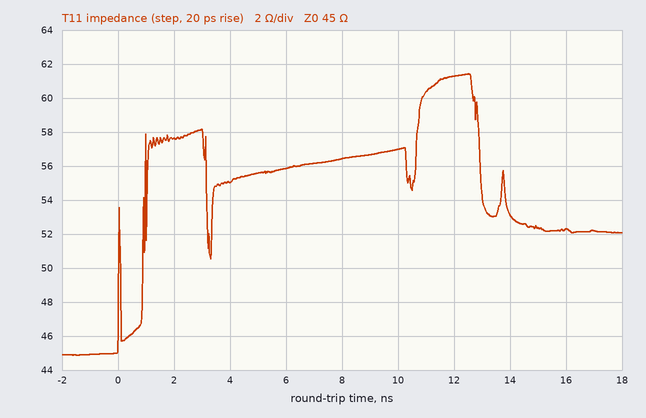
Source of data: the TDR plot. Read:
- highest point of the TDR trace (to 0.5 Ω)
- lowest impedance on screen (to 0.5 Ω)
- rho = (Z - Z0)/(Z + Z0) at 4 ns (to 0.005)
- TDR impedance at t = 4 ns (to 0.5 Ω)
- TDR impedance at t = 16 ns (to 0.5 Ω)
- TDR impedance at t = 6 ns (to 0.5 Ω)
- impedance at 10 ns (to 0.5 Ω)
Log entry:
61.5 Ω
45.0 Ω
+0.100
55.0 Ω
52.5 Ω
56.0 Ω
57.0 Ω
